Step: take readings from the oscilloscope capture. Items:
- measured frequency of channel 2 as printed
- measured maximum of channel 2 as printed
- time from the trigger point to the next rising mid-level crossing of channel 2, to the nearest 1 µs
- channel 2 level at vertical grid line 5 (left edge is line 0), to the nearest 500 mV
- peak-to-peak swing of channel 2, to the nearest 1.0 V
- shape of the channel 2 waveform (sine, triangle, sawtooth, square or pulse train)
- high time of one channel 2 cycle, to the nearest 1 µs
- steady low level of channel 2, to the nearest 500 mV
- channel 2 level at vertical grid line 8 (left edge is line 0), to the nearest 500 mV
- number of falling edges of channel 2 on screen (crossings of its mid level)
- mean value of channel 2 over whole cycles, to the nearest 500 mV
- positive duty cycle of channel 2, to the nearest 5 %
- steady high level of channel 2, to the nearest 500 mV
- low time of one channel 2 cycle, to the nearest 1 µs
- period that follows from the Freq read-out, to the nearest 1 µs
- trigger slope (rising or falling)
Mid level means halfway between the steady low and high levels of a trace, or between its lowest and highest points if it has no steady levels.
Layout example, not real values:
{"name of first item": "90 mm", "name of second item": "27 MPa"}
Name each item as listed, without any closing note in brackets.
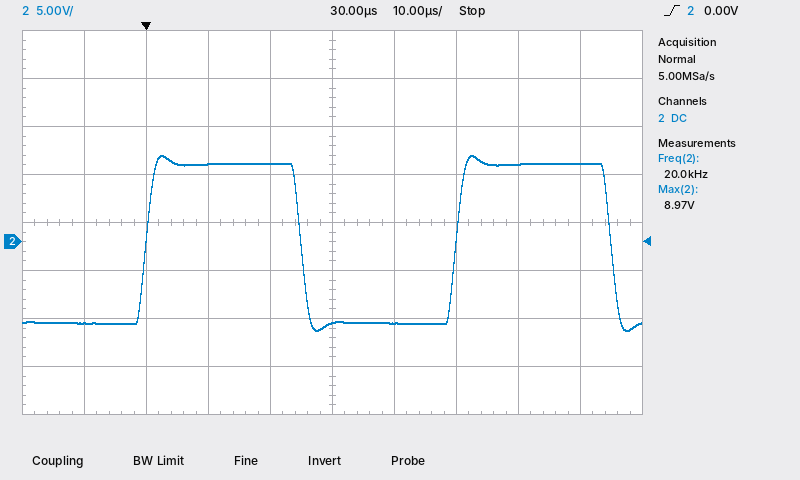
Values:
{"measured frequency of channel 2 as printed": "20.0 kHz", "measured maximum of channel 2 as printed": "8.97 V", "time from the trigger point to the next rising mid-level crossing of channel 2, to the nearest 1 µs": "50 µs", "channel 2 level at vertical grid line 5 (left edge is line 0), to the nearest 500 mV": "-8.5 V", "peak-to-peak swing of channel 2, to the nearest 1.0 V": "18.0 V", "shape of the channel 2 waveform": "square", "high time of one channel 2 cycle, to the nearest 1 µs": "25 µs", "steady low level of channel 2, to the nearest 500 mV": "-8.5 V", "channel 2 level at vertical grid line 8 (left edge is line 0), to the nearest 500 mV": "8.0 V", "number of falling edges of channel 2 on screen": "2", "mean value of channel 2 over whole cycles, to the nearest 500 mV": "0.0 V", "positive duty cycle of channel 2, to the nearest 5 %": "50 %", "steady high level of channel 2, to the nearest 500 mV": "8.0 V", "low time of one channel 2 cycle, to the nearest 1 µs": "25 µs", "period that follows from the Freq read-out, to the nearest 1 µs": "50 µs", "trigger slope": "rising"}
